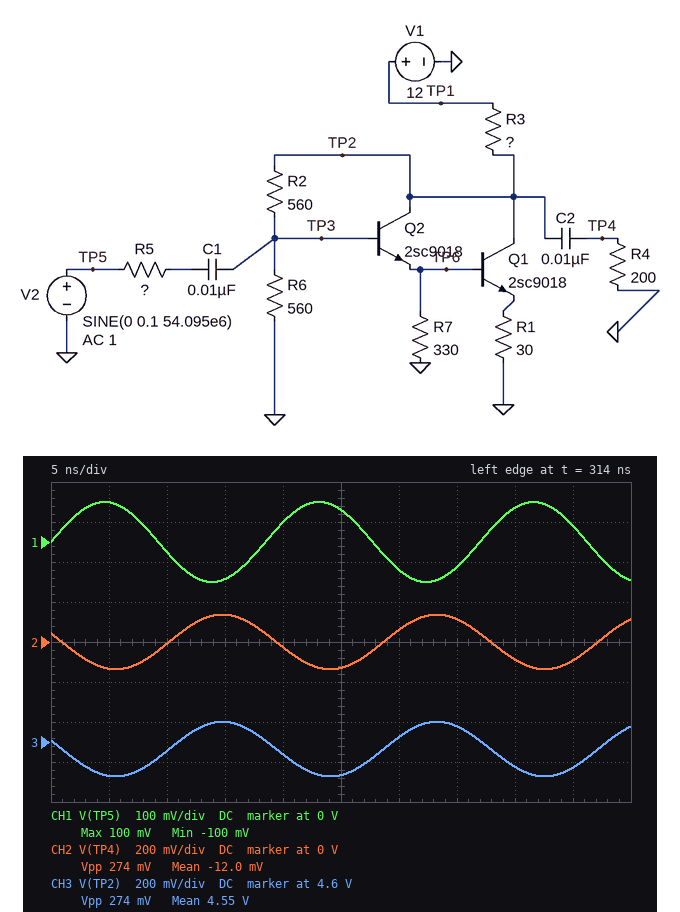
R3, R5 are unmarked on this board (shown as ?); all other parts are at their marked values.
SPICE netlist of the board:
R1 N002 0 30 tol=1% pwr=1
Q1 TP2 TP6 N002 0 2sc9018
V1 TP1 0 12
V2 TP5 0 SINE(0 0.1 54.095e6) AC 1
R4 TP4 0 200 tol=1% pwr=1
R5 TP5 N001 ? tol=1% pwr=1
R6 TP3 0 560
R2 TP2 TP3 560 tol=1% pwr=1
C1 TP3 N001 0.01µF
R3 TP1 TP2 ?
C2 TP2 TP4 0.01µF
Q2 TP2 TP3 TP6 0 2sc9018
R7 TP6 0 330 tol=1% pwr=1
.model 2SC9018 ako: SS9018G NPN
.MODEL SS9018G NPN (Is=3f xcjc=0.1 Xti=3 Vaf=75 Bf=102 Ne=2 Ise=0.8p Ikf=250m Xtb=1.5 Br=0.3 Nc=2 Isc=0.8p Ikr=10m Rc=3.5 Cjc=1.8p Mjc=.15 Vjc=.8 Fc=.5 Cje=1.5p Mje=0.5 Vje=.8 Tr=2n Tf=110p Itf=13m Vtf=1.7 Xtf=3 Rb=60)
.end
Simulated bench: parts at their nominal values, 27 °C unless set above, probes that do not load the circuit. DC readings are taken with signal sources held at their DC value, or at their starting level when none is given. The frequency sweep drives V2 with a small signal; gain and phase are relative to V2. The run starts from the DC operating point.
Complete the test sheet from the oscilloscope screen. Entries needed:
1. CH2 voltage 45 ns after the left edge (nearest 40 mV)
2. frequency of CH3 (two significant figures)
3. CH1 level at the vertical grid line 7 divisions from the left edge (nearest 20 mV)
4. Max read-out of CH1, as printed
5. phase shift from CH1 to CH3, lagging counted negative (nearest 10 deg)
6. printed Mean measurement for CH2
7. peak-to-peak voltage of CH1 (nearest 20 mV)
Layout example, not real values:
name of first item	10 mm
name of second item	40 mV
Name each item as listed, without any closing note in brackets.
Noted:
CH2 voltage 45 ns after the left edge	-80 mV
frequency of CH3	54 MHz
CH1 level at the vertical grid line 7 divisions from the left edge	-60 mV
Max read-out of CH1, as printed	100 mV
phase shift from CH1 to CH3, lagging counted negative	160 deg
printed Mean measurement for CH2	-12.0 mV
peak-to-peak voltage of CH1	200 mV
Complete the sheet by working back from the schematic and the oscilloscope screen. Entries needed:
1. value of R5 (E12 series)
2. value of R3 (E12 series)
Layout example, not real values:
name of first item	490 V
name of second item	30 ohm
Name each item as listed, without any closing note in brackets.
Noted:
value of R5	120 Ω
value of R3	220 Ω
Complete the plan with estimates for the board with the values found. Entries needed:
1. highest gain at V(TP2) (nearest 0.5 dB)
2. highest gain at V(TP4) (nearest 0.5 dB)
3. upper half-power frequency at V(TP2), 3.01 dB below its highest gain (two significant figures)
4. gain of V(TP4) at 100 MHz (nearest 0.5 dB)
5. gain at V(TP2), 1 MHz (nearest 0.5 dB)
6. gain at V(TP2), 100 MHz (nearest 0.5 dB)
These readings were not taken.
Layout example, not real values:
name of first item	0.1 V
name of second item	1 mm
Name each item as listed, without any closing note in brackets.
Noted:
highest gain at V(TP2)	3.0 dB
highest gain at V(TP4)	3.0 dB
upper half-power frequency at V(TP2), 3.01 dB below its highest gain	270 MHz
gain of V(TP4) at 100 MHz	2.5 dB
gain at V(TP2), 1 MHz	3.0 dB
gain at V(TP2), 100 MHz	2.5 dB
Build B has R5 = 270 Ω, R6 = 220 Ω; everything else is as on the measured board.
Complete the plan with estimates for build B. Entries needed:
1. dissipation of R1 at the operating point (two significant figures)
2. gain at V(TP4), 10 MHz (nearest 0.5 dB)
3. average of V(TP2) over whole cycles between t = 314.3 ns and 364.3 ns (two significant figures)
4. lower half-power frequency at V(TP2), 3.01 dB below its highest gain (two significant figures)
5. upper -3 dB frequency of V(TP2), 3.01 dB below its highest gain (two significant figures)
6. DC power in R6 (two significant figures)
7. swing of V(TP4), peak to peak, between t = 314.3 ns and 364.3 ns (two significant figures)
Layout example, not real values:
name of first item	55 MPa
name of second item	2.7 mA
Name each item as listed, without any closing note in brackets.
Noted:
dissipation of R1 at the operating point	4.8 mW
gain at V(TP4), 10 MHz	-3.5 dB
average of V(TP2) over whole cycles between t = 314.3 ns and 364.3 ns	6.6 V
lower half-power frequency at V(TP2), 3.01 dB below its highest gain	30 kHz
upper -3 dB frequency of V(TP2), 3.01 dB below its highest gain	330 MHz
DC power in R6	16 mW
swing of V(TP4), peak to peak, between t = 314.3 ns and 364.3 ns	130 mV
